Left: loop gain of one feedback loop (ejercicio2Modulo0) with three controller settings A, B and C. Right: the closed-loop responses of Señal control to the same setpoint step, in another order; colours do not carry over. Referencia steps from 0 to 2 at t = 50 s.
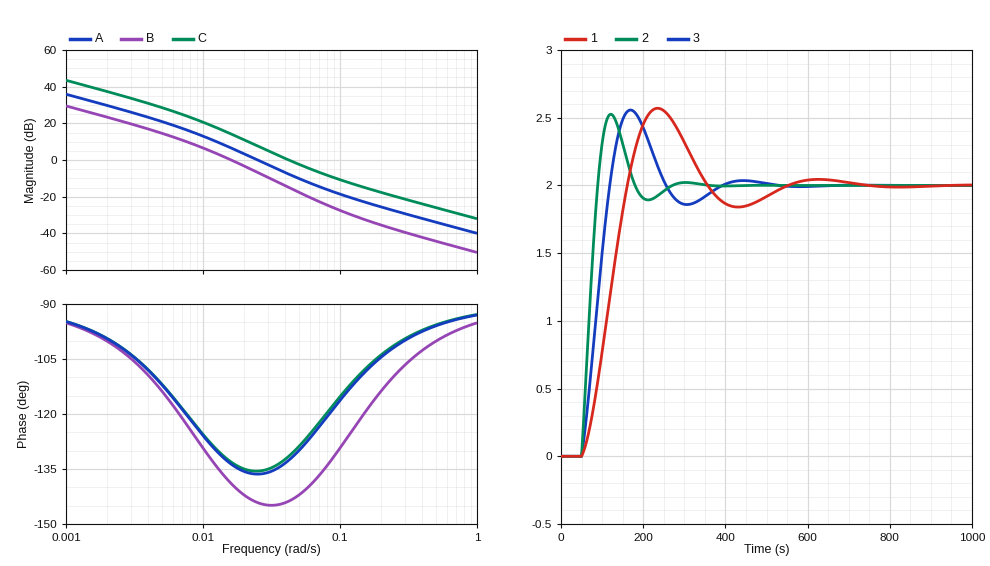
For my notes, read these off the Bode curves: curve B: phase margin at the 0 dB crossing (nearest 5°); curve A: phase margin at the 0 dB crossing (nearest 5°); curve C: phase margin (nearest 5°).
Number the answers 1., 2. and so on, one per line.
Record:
1. 40°
2. 45°
3. 50°
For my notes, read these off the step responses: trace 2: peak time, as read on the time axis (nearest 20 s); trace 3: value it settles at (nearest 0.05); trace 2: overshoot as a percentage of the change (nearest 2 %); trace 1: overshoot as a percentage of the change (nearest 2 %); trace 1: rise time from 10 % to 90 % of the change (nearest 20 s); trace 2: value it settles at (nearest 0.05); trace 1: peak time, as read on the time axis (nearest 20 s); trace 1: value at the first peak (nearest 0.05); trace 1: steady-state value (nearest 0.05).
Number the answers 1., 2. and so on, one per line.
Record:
1. 120 s
2. 2.00
3. 26 %
4. 28 %
5. 80 s
6. 2.00
7. 240 s
8. 2.55
9. 2.00
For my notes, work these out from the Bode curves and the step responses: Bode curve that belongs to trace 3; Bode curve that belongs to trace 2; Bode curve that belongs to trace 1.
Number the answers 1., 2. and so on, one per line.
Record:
1. A
2. C
3. B
